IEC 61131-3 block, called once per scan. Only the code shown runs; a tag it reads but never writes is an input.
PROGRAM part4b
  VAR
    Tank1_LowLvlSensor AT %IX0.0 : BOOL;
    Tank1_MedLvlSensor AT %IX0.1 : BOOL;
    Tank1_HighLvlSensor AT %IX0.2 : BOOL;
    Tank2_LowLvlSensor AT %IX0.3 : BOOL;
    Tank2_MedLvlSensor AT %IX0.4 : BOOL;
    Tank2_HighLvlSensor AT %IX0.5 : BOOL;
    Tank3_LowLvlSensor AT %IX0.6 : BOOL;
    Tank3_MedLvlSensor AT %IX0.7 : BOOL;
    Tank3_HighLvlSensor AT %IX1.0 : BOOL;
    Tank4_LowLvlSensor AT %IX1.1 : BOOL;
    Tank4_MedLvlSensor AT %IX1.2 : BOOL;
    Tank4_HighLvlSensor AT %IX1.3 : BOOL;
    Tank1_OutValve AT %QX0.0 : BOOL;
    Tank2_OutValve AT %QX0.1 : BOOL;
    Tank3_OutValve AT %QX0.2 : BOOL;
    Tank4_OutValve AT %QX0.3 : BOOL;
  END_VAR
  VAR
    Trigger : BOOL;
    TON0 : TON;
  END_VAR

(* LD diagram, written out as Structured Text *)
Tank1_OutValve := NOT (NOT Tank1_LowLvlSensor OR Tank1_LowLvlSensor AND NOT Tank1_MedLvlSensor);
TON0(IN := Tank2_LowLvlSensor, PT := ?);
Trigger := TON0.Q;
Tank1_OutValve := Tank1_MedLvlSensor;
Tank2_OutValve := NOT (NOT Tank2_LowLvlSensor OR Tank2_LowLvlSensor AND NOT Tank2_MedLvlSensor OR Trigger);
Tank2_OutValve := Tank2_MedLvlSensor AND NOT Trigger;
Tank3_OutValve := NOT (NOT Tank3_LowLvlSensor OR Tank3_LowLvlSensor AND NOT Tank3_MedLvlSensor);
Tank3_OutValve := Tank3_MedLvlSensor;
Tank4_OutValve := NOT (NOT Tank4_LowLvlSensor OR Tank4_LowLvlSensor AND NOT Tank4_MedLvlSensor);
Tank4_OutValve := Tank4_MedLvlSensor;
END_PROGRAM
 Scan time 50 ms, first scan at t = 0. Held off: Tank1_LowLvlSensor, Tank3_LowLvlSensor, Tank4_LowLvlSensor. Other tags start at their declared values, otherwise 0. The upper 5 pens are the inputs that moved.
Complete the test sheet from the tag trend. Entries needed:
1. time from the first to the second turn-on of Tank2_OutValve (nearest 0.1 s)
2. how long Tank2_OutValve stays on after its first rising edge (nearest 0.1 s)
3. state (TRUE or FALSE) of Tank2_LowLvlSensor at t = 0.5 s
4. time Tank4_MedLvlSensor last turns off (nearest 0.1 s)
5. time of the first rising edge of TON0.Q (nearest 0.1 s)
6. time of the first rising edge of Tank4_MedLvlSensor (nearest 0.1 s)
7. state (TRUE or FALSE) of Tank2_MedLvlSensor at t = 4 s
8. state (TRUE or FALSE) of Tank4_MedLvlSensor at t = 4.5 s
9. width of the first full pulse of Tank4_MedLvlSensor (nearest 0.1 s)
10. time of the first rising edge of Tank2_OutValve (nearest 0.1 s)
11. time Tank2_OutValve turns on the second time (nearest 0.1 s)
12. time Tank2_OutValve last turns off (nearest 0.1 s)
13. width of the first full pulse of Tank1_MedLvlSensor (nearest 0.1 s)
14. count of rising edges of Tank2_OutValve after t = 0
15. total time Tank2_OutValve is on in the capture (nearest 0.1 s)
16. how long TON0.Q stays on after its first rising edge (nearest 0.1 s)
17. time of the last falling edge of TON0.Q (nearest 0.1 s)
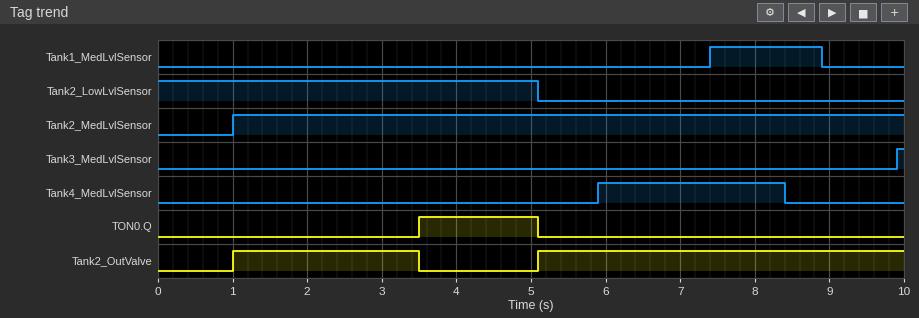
4.1 s
2.5 s
TRUE
8.4 s
3.5 s
5.9 s
TRUE
FALSE
2.5 s
1.0 s
5.1 s
3.5 s
1.5 s
2
7.4 s
1.6 s
5.1 s
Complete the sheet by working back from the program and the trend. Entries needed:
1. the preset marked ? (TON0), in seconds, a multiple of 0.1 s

3.5 s
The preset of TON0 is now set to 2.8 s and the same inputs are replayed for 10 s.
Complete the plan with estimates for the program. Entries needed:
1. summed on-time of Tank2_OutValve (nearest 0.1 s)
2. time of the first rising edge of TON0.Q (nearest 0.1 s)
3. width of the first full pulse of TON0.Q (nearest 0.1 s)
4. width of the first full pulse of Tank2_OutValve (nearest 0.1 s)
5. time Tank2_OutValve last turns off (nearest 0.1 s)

6.7 s
2.8 s
2.3 s
1.8 s
2.8 s
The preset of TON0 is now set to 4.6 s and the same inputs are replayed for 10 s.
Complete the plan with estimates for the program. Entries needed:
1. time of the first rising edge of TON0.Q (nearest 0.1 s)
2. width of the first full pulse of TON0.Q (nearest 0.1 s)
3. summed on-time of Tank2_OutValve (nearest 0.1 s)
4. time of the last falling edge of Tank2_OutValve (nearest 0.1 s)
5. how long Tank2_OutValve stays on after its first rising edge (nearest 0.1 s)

4.6 s
0.5 s
8.5 s
4.6 s
3.6 s
